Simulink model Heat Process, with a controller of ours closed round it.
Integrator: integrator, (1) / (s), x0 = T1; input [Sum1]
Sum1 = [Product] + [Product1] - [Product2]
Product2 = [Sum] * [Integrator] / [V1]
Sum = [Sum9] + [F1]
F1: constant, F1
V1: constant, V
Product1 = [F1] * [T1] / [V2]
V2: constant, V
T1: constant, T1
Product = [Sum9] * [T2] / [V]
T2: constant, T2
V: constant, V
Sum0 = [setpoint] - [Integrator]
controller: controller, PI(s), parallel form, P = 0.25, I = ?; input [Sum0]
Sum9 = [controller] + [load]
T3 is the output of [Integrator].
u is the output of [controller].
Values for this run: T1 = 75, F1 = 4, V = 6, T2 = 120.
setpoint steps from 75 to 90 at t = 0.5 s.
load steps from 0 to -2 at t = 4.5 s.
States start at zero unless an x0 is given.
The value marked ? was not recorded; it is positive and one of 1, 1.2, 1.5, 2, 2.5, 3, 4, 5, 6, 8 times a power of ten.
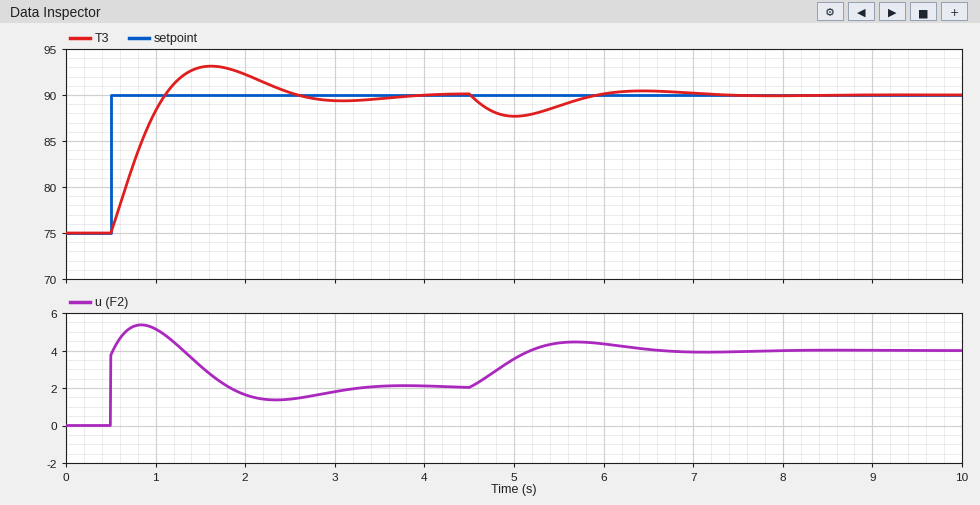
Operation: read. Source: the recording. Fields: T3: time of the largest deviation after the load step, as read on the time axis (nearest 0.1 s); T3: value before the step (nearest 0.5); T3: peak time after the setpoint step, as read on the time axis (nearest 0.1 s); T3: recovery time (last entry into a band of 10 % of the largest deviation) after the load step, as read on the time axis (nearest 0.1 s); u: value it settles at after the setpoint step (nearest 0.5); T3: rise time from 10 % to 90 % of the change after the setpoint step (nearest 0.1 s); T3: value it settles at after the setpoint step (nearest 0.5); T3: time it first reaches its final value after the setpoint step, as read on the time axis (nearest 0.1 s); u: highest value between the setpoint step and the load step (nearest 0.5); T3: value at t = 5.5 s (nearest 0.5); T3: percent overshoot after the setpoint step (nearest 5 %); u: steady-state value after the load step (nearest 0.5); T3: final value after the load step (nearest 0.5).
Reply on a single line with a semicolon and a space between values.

5.0 s; 75.0; 1.6 s; 6.9 s; 2.0; 0.5 s; 90.0; 1.1 s; 5.5; 89.0; 20 %; 4.0; 90.0
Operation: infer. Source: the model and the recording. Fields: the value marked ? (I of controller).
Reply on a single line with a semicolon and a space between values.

1.2
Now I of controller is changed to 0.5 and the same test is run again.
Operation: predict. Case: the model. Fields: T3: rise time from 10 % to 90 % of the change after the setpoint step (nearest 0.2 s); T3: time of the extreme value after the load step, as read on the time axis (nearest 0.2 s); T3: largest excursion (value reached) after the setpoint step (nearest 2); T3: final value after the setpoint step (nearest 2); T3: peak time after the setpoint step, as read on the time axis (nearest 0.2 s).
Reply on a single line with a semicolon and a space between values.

0.8 s; 5.2 s; 92; 90; 2.2 s
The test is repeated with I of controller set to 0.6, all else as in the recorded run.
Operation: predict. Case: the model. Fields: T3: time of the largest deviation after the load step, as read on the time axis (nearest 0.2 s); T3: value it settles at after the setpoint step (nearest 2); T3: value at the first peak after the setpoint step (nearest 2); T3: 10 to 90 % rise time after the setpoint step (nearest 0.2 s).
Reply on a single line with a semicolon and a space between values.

5.2 s; 90; 92; 0.6 s
